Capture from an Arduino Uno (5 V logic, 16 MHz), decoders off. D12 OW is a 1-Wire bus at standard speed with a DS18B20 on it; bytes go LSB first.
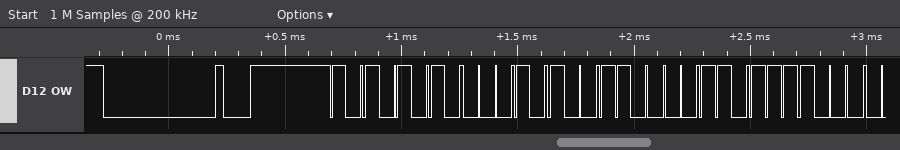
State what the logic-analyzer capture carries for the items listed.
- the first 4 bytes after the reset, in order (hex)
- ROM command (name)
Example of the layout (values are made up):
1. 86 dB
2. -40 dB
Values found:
1. 55 28 C3 1E
2. Match ROM
